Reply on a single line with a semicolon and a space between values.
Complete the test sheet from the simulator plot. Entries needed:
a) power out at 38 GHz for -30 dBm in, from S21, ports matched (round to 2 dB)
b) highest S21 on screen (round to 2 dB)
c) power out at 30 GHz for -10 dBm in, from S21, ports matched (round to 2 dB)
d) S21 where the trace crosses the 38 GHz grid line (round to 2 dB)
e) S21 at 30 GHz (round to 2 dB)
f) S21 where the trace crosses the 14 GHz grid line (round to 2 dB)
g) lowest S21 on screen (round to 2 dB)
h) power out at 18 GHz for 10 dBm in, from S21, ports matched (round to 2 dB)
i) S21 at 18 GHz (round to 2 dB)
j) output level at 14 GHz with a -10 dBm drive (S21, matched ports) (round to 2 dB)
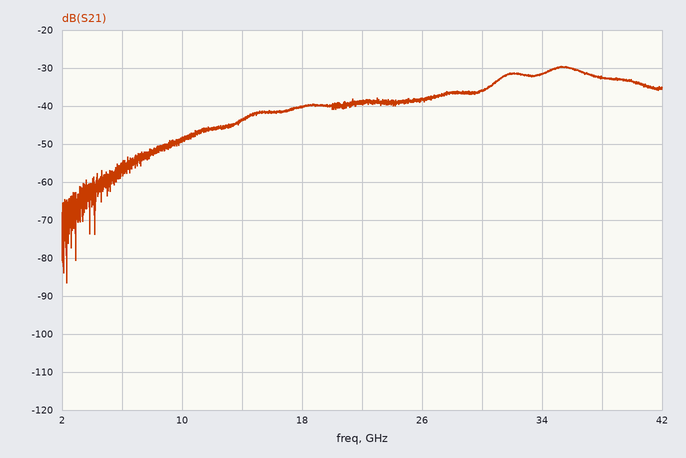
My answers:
-62 dBm; -30 dB; -46 dBm; -32 dB; -36 dB; -44 dB; -86 dB; -30 dBm; -40 dB; -54 dBm
